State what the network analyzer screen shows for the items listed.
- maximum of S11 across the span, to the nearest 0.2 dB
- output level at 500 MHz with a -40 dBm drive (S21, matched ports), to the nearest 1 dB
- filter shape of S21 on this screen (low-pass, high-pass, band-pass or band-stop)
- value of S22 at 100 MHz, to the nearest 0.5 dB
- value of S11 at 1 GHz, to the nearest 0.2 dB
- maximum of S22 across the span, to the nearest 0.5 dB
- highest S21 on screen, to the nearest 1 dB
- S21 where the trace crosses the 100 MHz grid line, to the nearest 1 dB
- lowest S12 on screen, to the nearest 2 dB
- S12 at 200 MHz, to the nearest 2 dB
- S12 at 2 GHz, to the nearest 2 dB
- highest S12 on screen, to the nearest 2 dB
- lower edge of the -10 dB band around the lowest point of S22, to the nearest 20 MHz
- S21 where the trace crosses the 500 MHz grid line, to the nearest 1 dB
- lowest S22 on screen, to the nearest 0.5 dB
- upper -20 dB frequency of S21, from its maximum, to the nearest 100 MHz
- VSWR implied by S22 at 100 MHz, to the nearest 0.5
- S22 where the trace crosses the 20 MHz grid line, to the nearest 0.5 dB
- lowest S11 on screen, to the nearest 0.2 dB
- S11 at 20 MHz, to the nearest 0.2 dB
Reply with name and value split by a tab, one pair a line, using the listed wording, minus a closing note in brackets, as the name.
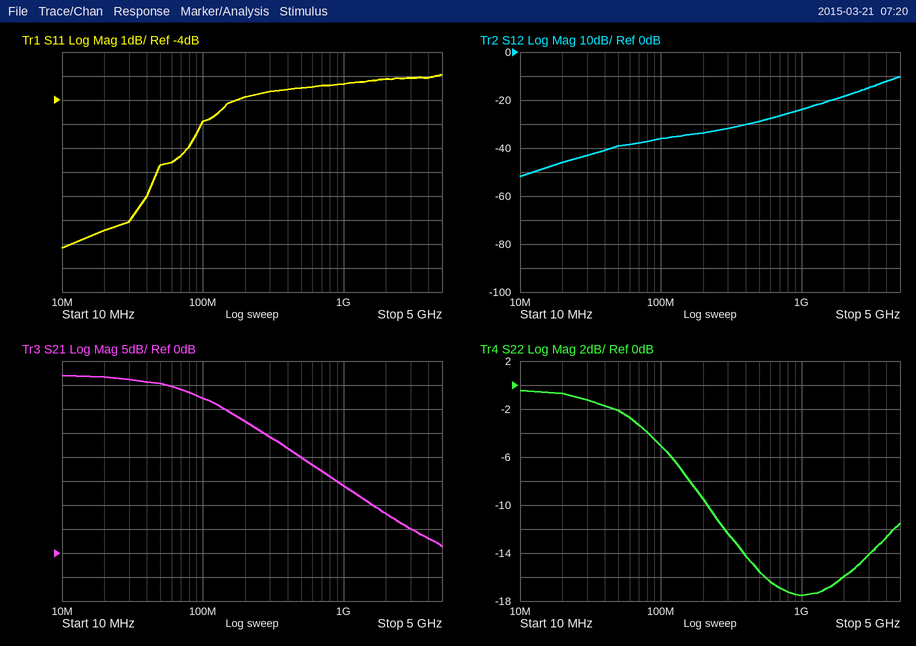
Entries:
maximum of S11 across the span, to the nearest 0.2 dB	-3.0 dB
output level at 500 MHz with a -40 dBm drive (S21, matched ports), to the nearest 1 dB	-20 dBm
filter shape of S21 on this screen	low-pass
value of S22 at 100 MHz, to the nearest 0.5 dB	-5.0 dB
value of S11 at 1 GHz, to the nearest 0.2 dB	-3.4 dB
maximum of S22 across the span, to the nearest 0.5 dB	-0.5 dB
highest S21 on screen, to the nearest 1 dB	37 dB
S21 where the trace crosses the 100 MHz grid line, to the nearest 1 dB	32 dB
lowest S12 on screen, to the nearest 2 dB	-52 dB
S12 at 200 MHz, to the nearest 2 dB	-34 dB
S12 at 2 GHz, to the nearest 2 dB	-18 dB
highest S12 on screen, to the nearest 2 dB	-10 dB
lower edge of the -10 dB band around the lowest point of S22, to the nearest 20 MHz	220 MHz
S21 where the trace crosses the 500 MHz grid line, to the nearest 1 dB	20 dB
lowest S22 on screen, to the nearest 0.5 dB	-17.5 dB
upper -20 dB frequency of S21, from its maximum, to the nearest 100 MHz	700 MHz
VSWR implied by S22 at 100 MHz, to the nearest 0.5	3.5
S22 where the trace crosses the 20 MHz grid line, to the nearest 0.5 dB	-0.5 dB
lowest S11 on screen, to the nearest 0.2 dB	-10.2 dB
S11 at 20 MHz, to the nearest 0.2 dB	-9.4 dB
